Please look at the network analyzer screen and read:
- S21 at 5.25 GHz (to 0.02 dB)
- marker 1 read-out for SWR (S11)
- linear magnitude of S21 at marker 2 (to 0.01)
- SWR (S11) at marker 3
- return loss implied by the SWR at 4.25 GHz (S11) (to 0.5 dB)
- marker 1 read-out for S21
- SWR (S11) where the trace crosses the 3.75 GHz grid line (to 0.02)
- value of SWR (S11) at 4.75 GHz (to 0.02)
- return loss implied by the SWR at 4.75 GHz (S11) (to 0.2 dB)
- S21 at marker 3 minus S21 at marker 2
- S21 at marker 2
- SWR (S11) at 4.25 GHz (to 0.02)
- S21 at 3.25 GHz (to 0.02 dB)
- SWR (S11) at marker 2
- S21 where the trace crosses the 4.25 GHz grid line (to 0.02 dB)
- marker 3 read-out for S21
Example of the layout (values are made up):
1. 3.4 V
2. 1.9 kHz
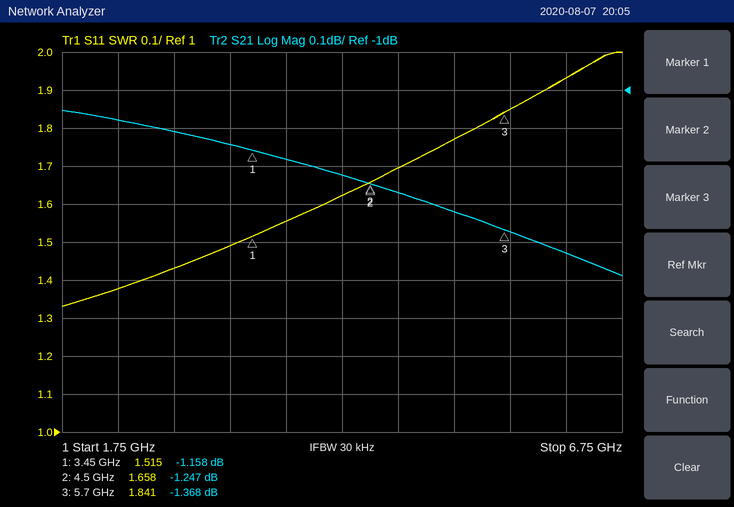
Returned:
1. -1.32 dB
2. 1.515
3. 0.87
4. 1.841
5. 12.5 dB
6. -1.158 dB
7. 1.56
8. 1.70
9. 11.8 dB
10. -0.121 dB
11. -1.247 dB
12. 1.62
13. -1.14 dB
14. 1.658
15. -1.22 dB
16. -1.368 dB
